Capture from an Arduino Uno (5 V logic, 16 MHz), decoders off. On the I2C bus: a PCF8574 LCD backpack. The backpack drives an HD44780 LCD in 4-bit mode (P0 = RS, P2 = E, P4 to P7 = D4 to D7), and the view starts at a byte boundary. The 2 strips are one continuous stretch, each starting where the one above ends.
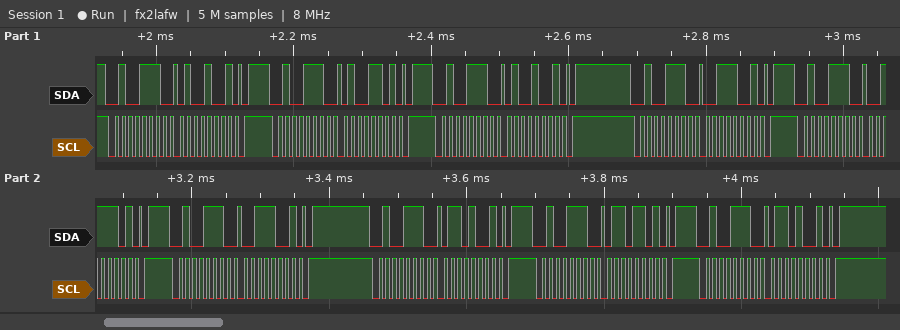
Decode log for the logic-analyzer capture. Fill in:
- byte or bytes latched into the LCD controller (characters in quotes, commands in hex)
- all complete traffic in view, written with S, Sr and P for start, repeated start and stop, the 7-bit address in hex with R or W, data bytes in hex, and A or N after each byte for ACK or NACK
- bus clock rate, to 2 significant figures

'C'
S 27W A 49 A P S 27W A 4D A P S 27W A 49 A P S 27W A 39 A P S 27W A 3D A P S 27W A 39 A P S 27W A 69 A P S 27W A 6D A P S 27W A 69 A P
100 kHz
